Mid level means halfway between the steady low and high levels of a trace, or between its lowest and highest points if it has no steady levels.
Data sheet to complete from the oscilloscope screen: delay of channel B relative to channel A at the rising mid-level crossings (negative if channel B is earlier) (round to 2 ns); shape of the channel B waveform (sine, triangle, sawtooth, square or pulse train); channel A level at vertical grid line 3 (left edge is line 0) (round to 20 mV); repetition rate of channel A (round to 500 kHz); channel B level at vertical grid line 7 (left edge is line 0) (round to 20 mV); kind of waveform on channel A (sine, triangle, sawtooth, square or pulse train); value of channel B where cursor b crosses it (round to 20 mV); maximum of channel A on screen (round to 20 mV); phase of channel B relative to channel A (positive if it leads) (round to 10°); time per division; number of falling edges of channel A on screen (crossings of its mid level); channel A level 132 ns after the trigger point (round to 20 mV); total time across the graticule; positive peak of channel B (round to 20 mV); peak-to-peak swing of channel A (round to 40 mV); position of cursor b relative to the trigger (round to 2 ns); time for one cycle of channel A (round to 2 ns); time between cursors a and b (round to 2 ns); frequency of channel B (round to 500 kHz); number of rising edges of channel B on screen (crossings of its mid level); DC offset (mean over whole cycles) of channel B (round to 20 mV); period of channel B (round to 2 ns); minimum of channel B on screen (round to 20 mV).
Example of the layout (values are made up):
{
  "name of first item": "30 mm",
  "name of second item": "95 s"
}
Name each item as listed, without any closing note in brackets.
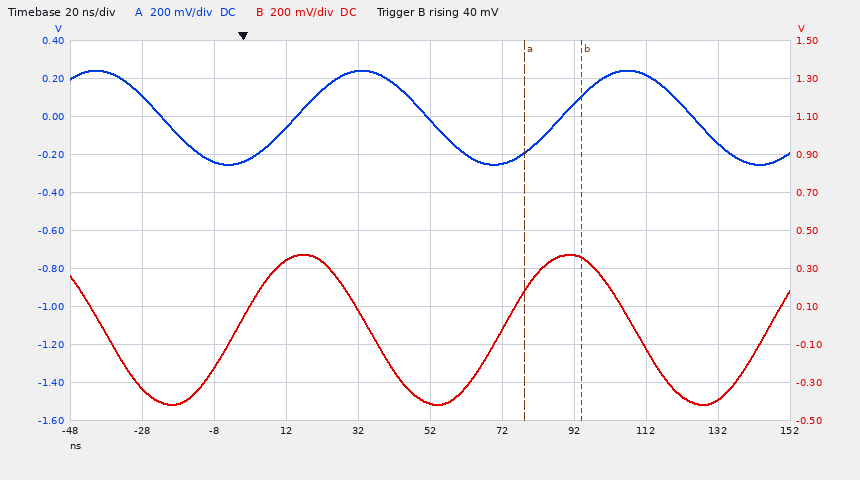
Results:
{
  "delay of channel B relative to channel A at the rising mid-level crossings (negative if channel B is earlier)": "-16 ns",
  "shape of the channel B waveform": "sine",
  "channel A level at vertical grid line 3 (left edge is line 0)": "-60 mV",
  "repetition rate of channel A": "13.5 MHz",
  "channel B level at vertical grid line 7 (left edge is line 0)": "380 mV",
  "kind of waveform on channel A": "sine",
  "value of channel B where cursor b crosses it": "360 mV",
  "maximum of channel A on screen": "240 mV",
  "phase of channel B relative to channel A (positive if it leads)": "+80°",
  "time per division": "20 ns",
  "number of falling edges of channel A on screen": "3",
  "channel A level 132 ns after the trigger point": "-140 mV",
  "total time across the graticule": "200 ns",
  "positive peak of channel B": "380 mV",
  "peak-to-peak swing of channel A": "480 mV",
  "position of cursor b relative to the trigger": "+94 ns",
  "time for one cycle of channel A": "74 ns",
  "time between cursors a and b": "16 ns",
  "frequency of channel B": "13.5 MHz",
  "number of rising edges of channel B on screen": "3",
  "DC offset (mean over whole cycles) of channel B": "-20 mV",
  "period of channel B": "74 ns",
  "minimum of channel B on screen": "-420 mV"
}
